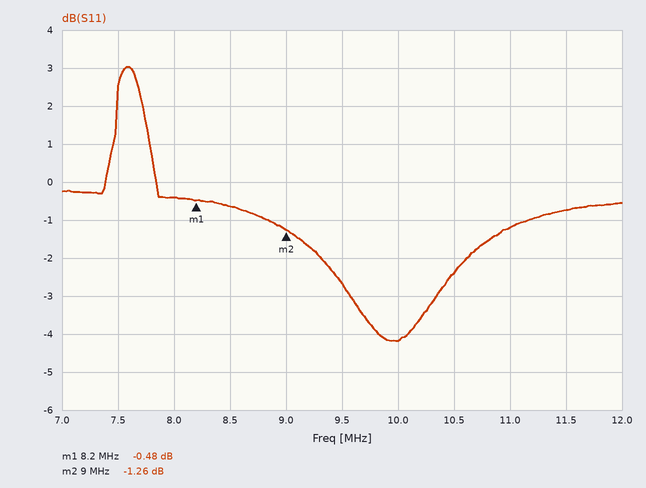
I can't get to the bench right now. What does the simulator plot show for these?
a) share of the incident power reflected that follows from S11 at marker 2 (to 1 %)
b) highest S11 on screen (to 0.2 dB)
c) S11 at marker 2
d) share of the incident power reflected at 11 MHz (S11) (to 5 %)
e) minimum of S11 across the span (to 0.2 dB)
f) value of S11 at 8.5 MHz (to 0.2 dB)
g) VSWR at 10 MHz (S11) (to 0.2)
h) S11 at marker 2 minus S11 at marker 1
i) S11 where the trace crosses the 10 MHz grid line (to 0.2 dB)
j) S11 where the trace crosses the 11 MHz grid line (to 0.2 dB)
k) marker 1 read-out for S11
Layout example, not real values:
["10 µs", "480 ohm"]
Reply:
["75 %", "3.0 dB", "-1.26 dB", "75 %", "-4.2 dB", "-0.6 dB", "4.2", "-0.78 dB", "-4.2 dB", "-1.2 dB", "-0.48 dB"]
